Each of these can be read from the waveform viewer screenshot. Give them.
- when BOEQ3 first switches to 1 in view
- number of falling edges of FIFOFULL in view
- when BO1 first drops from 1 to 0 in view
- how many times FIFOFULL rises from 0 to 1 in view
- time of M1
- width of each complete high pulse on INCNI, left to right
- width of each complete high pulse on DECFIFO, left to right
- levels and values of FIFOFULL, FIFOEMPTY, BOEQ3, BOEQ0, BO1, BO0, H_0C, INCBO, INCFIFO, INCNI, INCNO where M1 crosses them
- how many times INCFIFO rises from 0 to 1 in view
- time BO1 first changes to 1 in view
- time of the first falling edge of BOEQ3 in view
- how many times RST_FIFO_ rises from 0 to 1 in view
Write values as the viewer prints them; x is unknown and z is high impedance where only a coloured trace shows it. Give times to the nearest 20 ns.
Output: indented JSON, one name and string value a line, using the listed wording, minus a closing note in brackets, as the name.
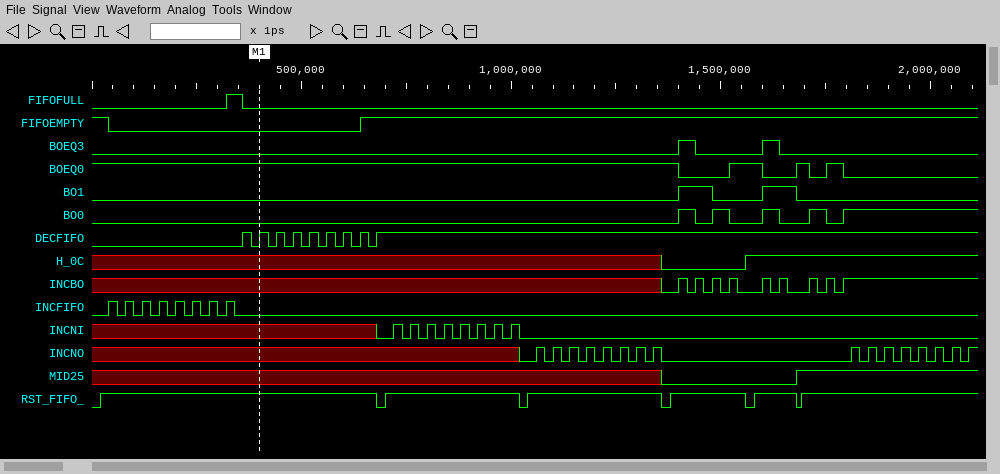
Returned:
{
  "when BOEQ3 first switches to 1 in view": "1400 ns",
  "number of falling edges of FIFOFULL in view": "1",
  "when BO1 first drops from 1 to 0 in view": "1480 ns",
  "how many times FIFOFULL rises from 0 to 1 in view": "1",
  "time of M1": "400 ns",
  "width of each complete high pulse on INCNI, left to right": "20 ns, 20 ns, 20 ns, 20 ns, 20 ns, 20 ns, 20 ns, 20 ns",
  "width of each complete high pulse on DECFIFO, left to right": "20 ns, 20 ns, 20 ns, 20 ns, 20 ns, 20 ns, 20 ns, 20 ns",
  "levels and values of FIFOFULL, FIFOEMPTY, BOEQ3, BOEQ0, BO1, BO0, H_0C, INCBO, INCFIFO, INCNI, INCNO where M1 crosses them": "FIFOFULL=0, FIFOEMPTY=0, BOEQ3=0, BOEQ0=1, BO1=0, BO0=0, H_0C=x, INCBO=x, INCFIFO=0, INCNI=x, INCNO=x",
  "how many times INCFIFO rises from 0 to 1 in view": "8",
  "time BO1 first changes to 1 in view": "1400 ns",
  "time of the first falling edge of BOEQ3 in view": "1440 ns",
  "how many times RST_FIFO_ rises from 0 to 1 in view": "6"
}
